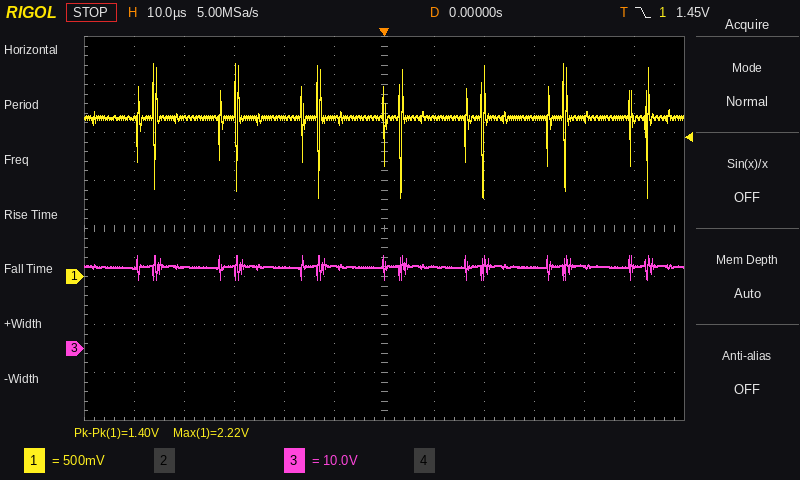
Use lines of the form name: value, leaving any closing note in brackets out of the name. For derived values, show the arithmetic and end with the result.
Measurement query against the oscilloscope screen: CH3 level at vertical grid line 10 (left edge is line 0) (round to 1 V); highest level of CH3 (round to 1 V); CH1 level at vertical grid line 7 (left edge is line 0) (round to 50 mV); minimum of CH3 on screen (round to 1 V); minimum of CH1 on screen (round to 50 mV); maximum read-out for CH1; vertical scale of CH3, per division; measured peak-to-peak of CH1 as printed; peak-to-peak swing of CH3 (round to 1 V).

CH3 level at vertical grid line 10 (left edge is line 0): 17 V
highest level of CH3: 19 V
CH1 level at vertical grid line 7 (left edge is line 0): 1.65 V
minimum of CH3 on screen: 14 V
minimum of CH1 on screen: 800 mV
maximum read-out for CH1: 2.22 V
vertical scale of CH3, per division: 10 V
measured peak-to-peak of CH1 as printed: 1.40 V
peak-to-peak swing of CH3: 19 V − (14 V) = 5 V
